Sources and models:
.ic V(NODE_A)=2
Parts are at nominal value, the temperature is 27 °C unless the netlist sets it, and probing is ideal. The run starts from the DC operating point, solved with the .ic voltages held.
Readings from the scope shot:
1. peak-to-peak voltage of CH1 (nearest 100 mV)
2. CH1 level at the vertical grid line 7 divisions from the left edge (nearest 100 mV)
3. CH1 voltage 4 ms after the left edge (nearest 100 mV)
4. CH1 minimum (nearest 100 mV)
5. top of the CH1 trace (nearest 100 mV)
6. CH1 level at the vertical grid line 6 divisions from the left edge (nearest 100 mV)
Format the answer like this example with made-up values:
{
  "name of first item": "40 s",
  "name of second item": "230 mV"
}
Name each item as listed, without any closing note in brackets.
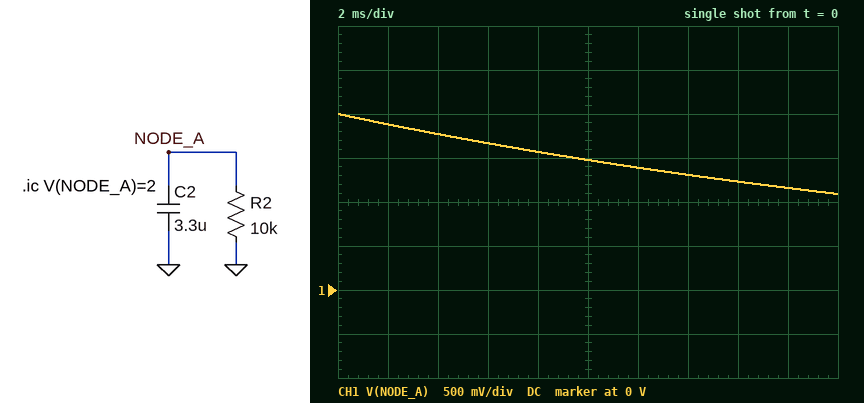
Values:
{
  "peak-to-peak voltage of CH1": "900 mV",
  "CH1 level at the vertical grid line 7 divisions from the left edge": "1.3 V",
  "CH1 voltage 4 ms after the left edge": "1.8 V",
  "CH1 minimum": "1.1 V",
  "top of the CH1 trace": "2.0 V",
  "CH1 level at the vertical grid line 6 divisions from the left edge": "1.4 V"
}
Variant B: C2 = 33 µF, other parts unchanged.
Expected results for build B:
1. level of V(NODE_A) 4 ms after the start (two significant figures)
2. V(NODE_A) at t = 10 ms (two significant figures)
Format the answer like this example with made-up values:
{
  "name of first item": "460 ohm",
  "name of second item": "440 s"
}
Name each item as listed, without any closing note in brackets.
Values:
{
  "level of V(NODE_A) 4 ms after the start": "2.0 V",
  "V(NODE_A) at t = 10 ms": "1.9 V"
}
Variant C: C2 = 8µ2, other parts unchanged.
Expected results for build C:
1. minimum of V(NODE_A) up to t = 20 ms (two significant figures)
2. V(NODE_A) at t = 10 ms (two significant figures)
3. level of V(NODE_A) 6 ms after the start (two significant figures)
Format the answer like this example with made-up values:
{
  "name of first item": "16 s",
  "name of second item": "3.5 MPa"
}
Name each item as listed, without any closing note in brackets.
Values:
{
  "minimum of V(NODE_A) up to t = 20 ms": "1.6 V",
  "V(NODE_A) at t = 10 ms": "1.8 V",
  "level of V(NODE_A) 6 ms after the start": "1.9 V"
}
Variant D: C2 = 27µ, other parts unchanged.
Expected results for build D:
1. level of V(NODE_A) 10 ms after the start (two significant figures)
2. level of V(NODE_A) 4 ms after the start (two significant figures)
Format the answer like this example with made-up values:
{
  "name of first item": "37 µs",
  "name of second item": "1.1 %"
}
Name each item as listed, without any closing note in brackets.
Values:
{
  "level of V(NODE_A) 10 ms after the start": "1.9 V",
  "level of V(NODE_A) 4 ms after the start": "2.0 V"
}
